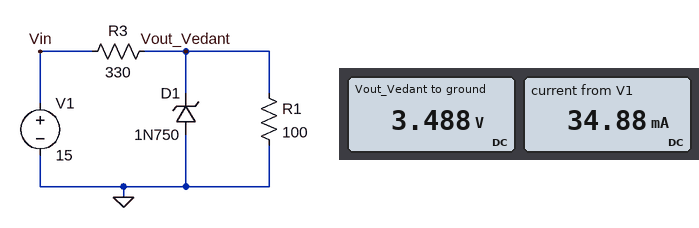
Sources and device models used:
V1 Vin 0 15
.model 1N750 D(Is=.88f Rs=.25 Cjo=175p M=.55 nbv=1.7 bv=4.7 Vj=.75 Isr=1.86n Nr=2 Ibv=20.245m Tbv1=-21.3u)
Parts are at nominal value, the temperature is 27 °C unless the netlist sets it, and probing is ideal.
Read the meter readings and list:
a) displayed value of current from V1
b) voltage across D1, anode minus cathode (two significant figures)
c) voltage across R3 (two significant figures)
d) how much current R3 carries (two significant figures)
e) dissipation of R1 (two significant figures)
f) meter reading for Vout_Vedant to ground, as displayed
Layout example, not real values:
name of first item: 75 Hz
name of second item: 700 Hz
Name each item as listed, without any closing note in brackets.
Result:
displayed value of current from V1: 34.88 mA
voltage across D1, anode minus cathode: -3.5 V
voltage across R3: 12 V
how much current R3 carries: 35 mA
dissipation of R1: 120 mW
meter reading for Vout_Vedant to ground, as displayed: 3.488 V
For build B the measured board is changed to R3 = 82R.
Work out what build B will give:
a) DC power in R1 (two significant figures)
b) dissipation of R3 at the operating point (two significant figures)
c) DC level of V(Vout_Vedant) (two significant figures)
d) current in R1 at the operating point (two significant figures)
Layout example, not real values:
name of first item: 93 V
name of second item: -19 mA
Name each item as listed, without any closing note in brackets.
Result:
DC power in R1: 230 mW
dissipation of R3 at the operating point: 1.3 W
DC level of V(Vout_Vedant): 4.8 V
current in R1 at the operating point: 48 mA
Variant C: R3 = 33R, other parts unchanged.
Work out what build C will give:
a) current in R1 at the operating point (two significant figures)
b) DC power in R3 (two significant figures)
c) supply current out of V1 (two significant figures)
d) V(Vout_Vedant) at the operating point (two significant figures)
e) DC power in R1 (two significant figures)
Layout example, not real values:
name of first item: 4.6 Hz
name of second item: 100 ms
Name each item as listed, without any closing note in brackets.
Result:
current in R1 at the operating point: 49 mA
DC power in R3: 3.1 W
supply current out of V1: 310 mA
V(Vout_Vedant) at the operating point: 4.9 V
DC power in R1: 240 mW
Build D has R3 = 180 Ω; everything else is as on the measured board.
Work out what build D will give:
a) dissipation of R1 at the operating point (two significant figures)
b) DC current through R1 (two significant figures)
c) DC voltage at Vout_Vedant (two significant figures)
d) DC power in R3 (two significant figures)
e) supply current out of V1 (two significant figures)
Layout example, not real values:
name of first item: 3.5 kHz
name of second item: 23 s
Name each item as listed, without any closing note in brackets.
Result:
dissipation of R1 at the operating point: 220 mW
DC current through R1: 47 mA
DC voltage at Vout_Vedant: 4.7 V
DC power in R3: 590 mW
supply current out of V1: 57 mA
